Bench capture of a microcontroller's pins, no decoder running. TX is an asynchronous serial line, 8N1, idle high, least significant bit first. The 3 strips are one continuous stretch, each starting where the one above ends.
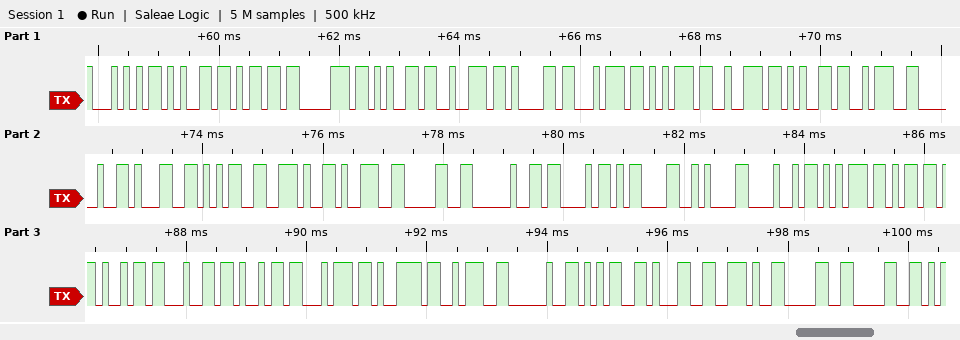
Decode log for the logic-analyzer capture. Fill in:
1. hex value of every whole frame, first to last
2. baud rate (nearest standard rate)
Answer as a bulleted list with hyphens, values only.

- 0x54 0x65 0x6D 0x70 0x65 0x72 0x61 0x74 0x75 0x72 0x65 0x3A 0x20 0x31 0x35 0x2E 0x39 0x30 0x20 0x43 0x0D 0x0A 0x48 0x75 0x6D 0x69 0x64 0x69 0x74 0x79 0x3A 0x20 0x35 0x31 0x2E 0x30 0x30
- 9600 baud
